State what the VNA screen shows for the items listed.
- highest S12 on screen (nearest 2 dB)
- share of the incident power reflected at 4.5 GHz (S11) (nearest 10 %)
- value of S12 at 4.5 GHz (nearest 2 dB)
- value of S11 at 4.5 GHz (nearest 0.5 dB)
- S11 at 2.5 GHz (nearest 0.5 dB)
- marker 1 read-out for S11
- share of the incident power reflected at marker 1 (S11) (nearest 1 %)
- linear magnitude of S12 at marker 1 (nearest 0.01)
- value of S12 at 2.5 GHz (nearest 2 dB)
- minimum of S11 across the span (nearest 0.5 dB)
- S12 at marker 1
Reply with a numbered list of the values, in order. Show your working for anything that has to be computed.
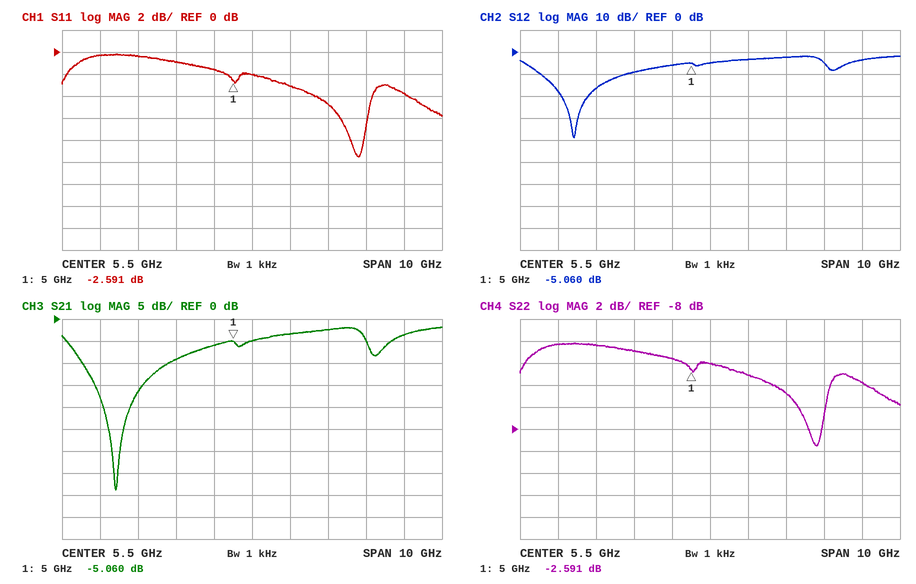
1. -2 dB
2. 10^(-1.5/10) ≈ 70.8 %, so 70 % to the nearest 10 %
3. -6 dB
4. -1.5 dB
5. -0.5 dB
6. -2.591 dB
7. 10^(-2.591/10) ≈ 55 %
8. 10^(-5.06/20) ≈ 0.56
9. -16 dB
10. -9.5 dB
11. -5.060 dB
